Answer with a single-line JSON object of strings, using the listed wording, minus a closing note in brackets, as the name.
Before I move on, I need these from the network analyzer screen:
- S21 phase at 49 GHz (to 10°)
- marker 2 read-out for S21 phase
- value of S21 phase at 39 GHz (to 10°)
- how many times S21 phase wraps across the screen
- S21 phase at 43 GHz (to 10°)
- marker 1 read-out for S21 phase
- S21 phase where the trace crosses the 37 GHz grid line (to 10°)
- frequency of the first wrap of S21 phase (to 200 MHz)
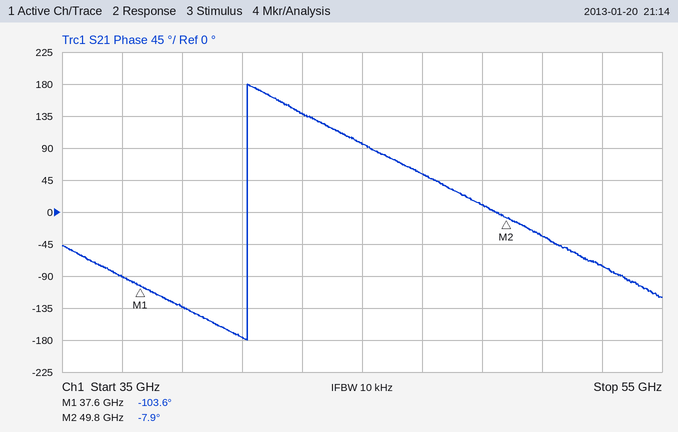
{"S21 phase at 49 GHz": "10°", "marker 2 read-out for S21 phase": "-7.9°", "value of S21 phase at 39 GHz": "-130°", "how many times S21 phase wraps across the screen": "1", "S21 phase at 43 GHz": "140°", "marker 1 read-out for S21 phase": "-103.6°", "S21 phase where the trace crosses the 37 GHz grid line": "-90°", "frequency of the first wrap of S21 phase": "41.2 GHz"}
